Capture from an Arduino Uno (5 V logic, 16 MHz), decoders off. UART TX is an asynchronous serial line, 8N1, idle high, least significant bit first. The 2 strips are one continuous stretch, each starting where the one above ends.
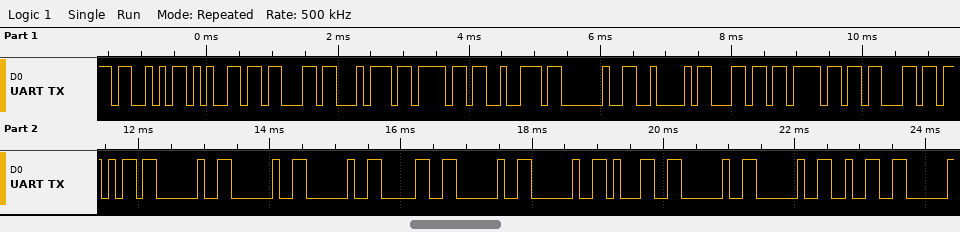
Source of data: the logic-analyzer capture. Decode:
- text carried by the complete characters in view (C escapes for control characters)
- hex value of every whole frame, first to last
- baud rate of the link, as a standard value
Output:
"Sector Block   0  1  2"
53 65 63 74 6F 72 20 42 6C 6F 63 6B 20 20 20 30 20 20 31 20 20 32
9600 baud
